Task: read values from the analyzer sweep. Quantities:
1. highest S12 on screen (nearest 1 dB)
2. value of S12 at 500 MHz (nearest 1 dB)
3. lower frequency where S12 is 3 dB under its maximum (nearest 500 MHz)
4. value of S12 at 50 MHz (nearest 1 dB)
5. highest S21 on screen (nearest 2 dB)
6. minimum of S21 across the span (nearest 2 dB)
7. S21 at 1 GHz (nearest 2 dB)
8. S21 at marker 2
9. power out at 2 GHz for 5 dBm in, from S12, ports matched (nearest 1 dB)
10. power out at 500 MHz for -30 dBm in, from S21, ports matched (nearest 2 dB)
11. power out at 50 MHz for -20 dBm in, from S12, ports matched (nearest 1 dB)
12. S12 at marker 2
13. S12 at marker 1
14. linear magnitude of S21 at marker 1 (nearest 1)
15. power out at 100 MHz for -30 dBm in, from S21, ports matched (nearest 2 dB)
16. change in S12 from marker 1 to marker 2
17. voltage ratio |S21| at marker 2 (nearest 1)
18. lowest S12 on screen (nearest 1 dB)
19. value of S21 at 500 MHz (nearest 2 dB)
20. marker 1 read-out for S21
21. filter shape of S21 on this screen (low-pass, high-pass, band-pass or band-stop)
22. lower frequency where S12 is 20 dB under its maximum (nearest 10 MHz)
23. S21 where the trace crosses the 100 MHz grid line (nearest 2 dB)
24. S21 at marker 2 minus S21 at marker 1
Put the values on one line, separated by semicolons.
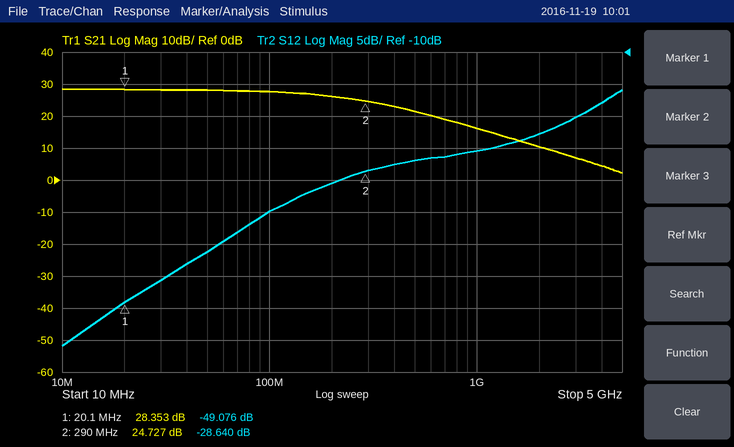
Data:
-16 dB; -27 dB; 3.5 GHz; -41 dB; 28 dB; 2 dB; 16 dB; 24.727 dB; -18 dBm; -8 dBm; -61 dBm; -28.640 dB; -49.076 dB; 26; -2 dBm; 20.436 dB; 17; -56 dB; 22 dB; 28.353 dB; low-pass; 90 MHz; 28 dB; -3.626 dB
